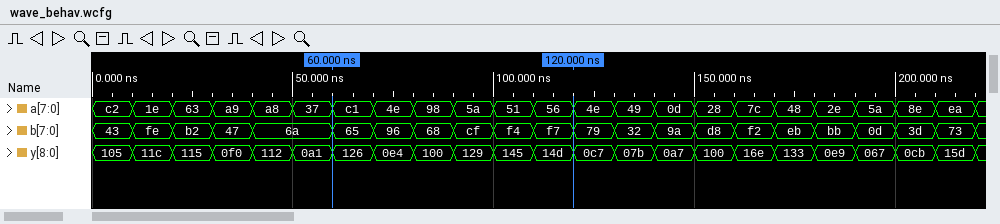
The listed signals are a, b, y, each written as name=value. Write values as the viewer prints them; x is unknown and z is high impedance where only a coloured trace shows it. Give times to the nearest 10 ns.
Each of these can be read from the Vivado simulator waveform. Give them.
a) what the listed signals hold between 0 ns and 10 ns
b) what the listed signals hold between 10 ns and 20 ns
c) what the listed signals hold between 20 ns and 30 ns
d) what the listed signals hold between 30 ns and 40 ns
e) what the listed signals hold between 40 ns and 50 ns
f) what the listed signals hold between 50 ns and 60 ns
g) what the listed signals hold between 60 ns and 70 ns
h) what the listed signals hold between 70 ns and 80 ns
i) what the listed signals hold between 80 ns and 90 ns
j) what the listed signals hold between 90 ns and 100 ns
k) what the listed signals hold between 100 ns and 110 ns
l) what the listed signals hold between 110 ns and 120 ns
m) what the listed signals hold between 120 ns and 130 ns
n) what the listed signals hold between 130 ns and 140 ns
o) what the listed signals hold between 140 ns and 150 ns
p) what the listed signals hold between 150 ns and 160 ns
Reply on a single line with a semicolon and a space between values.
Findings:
a=c2, b=43, y=105; a=1e, b=fe, y=11c; a=63, b=b2, y=115; a=a9, b=47, y=0f0; a=a8, b=6a, y=112; a=37, b=6a, y=0a1; a=c1, b=65, y=126; a=4e, b=96, y=0e4; a=98, b=68, y=100; a=5a, b=cf, y=129; a=51, b=f4, y=145; a=56, b=f7, y=14d; a=4e, b=79, y=0c7; a=49, b=32, y=07b; a=0d, b=9a, y=0a7; a=28, b=d8, y=100
